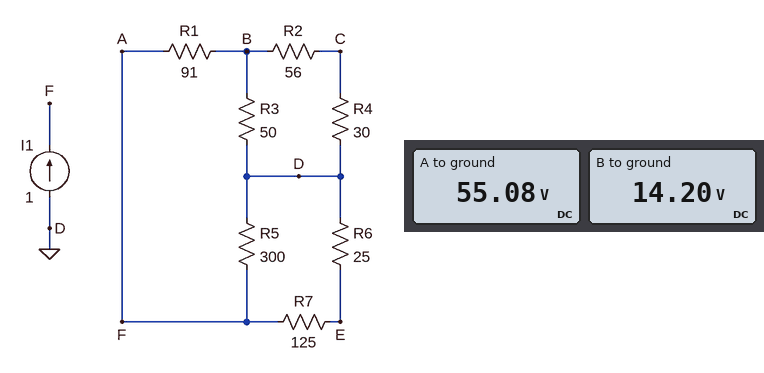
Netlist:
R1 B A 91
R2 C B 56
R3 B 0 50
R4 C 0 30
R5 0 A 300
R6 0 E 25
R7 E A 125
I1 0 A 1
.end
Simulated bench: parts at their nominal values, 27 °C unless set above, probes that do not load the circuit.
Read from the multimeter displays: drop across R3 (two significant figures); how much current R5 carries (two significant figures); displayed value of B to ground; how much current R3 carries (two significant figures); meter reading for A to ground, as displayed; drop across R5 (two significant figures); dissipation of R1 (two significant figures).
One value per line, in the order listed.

14 V
180 mA
14.20 V
280 mA
55.08 V
55 V
18 W
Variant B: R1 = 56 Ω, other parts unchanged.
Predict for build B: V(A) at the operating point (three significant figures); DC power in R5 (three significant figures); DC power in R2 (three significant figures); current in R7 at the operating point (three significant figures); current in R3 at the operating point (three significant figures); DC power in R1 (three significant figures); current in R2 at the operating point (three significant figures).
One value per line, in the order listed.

46.7 V
7.27 W
2.15 W
311 mA
337 mA
15.9 W
196 mA
